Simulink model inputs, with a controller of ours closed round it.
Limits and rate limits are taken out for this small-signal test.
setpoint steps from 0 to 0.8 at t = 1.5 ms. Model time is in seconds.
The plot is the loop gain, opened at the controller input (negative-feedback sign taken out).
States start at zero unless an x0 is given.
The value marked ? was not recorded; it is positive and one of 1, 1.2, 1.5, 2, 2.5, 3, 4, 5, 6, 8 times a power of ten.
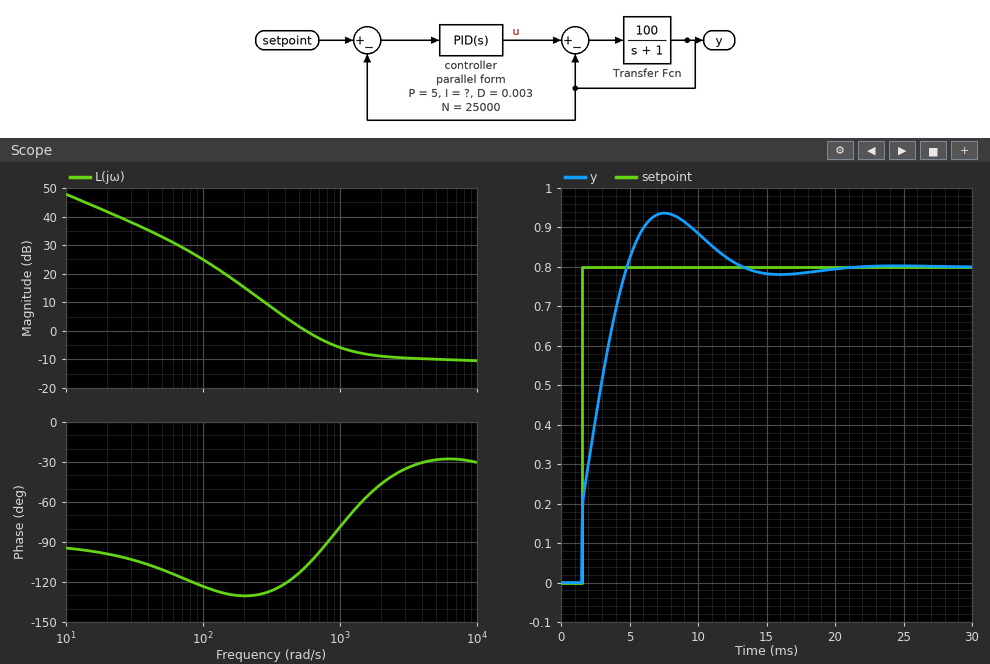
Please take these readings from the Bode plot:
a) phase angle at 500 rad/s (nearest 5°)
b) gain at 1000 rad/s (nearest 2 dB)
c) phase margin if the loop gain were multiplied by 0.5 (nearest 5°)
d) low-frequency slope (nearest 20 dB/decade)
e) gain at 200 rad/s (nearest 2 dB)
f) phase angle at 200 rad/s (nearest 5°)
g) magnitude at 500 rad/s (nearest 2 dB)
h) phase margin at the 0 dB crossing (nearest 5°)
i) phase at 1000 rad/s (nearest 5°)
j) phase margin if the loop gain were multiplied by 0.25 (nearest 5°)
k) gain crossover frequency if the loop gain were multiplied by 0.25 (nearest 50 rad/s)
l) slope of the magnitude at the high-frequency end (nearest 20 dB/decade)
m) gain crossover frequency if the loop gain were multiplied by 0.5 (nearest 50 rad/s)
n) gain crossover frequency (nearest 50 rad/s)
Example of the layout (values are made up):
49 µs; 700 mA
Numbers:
-115°; -6 dB; 55°; -20 dB/decade; 16 dB; -130°; 2 dB; 70°; -80°; 50°; 250 rad/s; 0 dB/decade; 350 rad/s; 550 rad/s
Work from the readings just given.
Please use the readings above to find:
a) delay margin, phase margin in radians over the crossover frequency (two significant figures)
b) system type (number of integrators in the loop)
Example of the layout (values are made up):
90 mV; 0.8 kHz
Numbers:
0.0022 s; 1
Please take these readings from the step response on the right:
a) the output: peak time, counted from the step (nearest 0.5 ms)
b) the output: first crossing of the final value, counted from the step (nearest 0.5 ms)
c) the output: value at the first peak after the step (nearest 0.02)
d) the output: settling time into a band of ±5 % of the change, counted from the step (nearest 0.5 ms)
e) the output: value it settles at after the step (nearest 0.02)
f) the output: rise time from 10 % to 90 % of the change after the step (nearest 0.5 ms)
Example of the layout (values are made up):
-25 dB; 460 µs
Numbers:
6.0 ms; 3.5 ms; 0.94; 10.0 ms; 0.80; 2.5 ms
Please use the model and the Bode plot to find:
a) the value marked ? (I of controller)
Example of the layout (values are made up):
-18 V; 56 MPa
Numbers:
2500
